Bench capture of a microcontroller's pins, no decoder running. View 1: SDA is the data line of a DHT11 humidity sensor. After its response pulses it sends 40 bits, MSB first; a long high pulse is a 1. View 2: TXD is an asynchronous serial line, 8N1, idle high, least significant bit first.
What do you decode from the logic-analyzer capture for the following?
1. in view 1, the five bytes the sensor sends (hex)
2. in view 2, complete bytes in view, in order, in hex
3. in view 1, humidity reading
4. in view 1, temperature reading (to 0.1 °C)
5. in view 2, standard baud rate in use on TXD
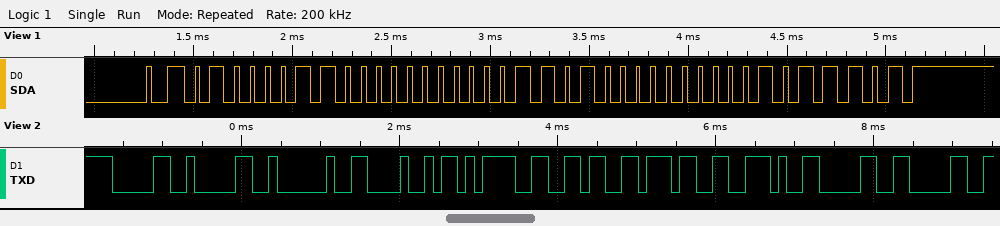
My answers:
43 00 1A 00 5D
0x30 0x30 0x20 0x48 0x3D 0x36 0x37 0x2E 0x30 0x30
67 %
26.0 °C
9600 baud
